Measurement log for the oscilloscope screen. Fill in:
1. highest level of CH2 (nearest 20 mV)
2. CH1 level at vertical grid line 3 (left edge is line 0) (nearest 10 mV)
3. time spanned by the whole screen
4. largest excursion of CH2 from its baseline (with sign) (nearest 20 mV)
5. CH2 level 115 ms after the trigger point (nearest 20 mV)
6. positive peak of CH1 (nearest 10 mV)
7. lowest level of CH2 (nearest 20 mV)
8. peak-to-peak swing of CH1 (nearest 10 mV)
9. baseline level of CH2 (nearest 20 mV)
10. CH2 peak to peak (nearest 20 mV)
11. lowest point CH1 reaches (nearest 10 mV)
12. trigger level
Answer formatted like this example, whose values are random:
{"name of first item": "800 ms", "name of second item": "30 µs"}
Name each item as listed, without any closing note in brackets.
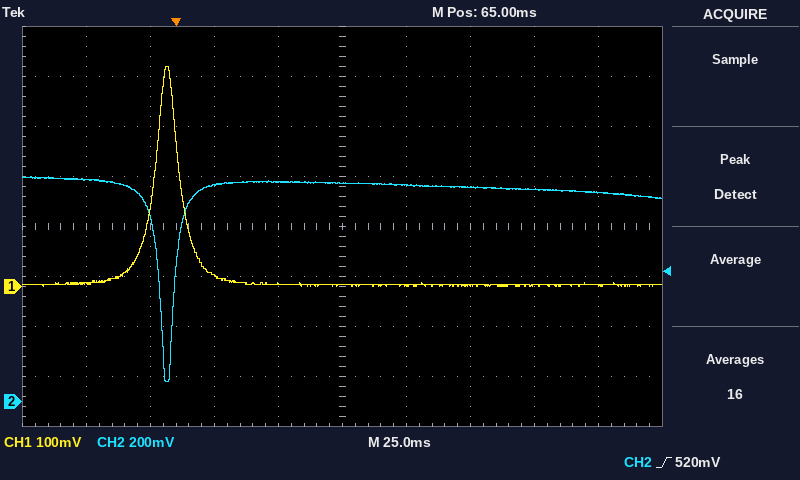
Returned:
{"highest level of CH2": "900 mV", "CH1 level at vertical grid line 3 (left edge is line 0)": "20 mV", "time spanned by the whole screen": "250 ms", "largest excursion of CH2 from its baseline (with sign)": "-780 mV", "CH2 level 115 ms after the trigger point": "860 mV", "positive peak of CH1": "440 mV", "lowest level of CH2": "80 mV", "peak-to-peak swing of CH1": "440 mV", "baseline level of CH2": "860 mV", "CH2 peak to peak": "820 mV", "lowest point CH1 reaches": "0 mV", "trigger level": "520 mV"}
